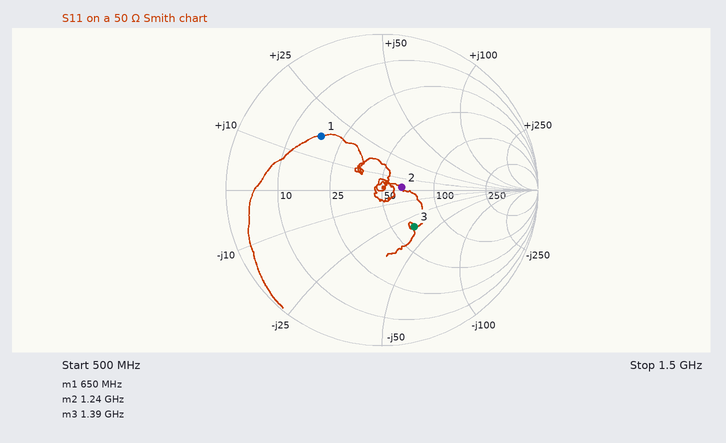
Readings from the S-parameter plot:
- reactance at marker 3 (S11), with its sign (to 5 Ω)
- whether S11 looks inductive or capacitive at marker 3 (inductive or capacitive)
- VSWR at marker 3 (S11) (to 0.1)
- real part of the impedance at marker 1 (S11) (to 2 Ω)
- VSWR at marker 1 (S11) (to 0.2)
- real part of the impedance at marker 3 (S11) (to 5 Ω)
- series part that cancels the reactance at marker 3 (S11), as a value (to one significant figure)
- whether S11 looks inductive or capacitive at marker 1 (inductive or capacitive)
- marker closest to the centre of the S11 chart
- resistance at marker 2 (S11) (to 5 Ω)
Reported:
-35 Ω
capacitive
1.9
18 Ω
3.2
65 Ω
4 nH
inductive
marker 2
65 Ω
